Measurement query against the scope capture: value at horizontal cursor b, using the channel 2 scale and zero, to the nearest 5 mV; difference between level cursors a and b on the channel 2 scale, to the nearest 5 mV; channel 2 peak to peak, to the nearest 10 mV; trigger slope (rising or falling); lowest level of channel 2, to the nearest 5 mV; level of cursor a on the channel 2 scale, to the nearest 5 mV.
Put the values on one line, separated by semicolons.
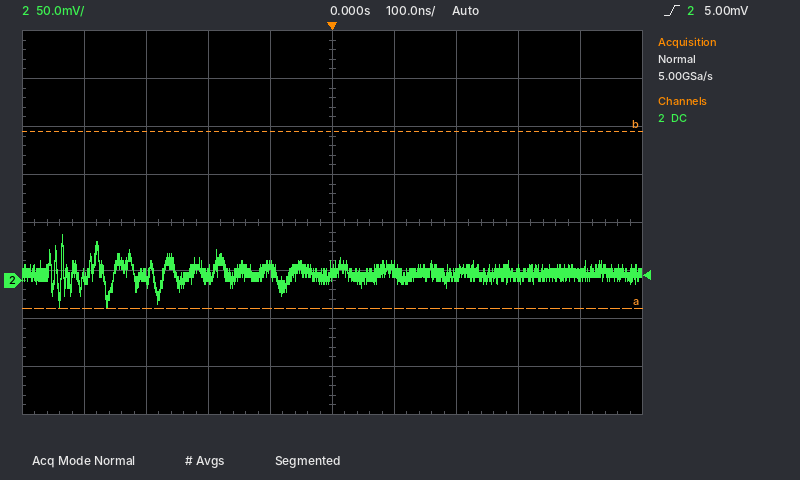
155 mV; 185 mV; 80 mV; rising; -30 mV; -30 mV
